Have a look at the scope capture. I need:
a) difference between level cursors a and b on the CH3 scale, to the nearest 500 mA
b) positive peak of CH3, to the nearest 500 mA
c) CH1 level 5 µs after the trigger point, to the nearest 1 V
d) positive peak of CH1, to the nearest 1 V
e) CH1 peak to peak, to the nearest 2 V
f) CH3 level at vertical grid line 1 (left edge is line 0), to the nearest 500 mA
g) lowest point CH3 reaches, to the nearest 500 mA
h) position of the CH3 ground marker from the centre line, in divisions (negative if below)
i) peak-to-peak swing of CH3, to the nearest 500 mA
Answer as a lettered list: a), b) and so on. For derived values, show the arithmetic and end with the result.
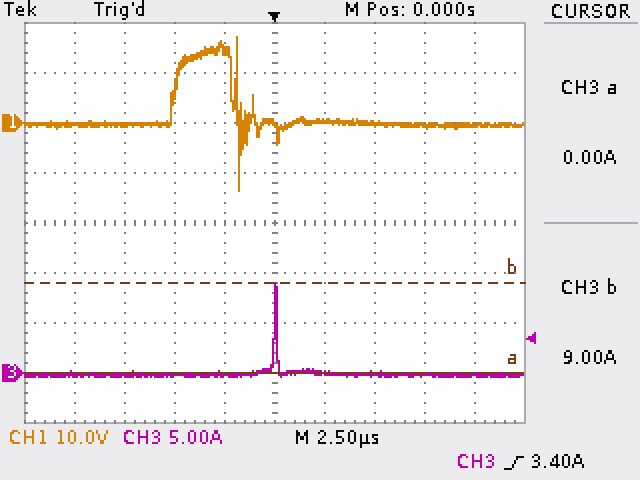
a) 9.0 A
b) 9.0 A
c) 0 V
d) 17 V
e) 30 V
f) 0.0 A
g) -500 mA
h) -3.0 div
i) 9.0 A − (-500 mA) = 9.5 A
